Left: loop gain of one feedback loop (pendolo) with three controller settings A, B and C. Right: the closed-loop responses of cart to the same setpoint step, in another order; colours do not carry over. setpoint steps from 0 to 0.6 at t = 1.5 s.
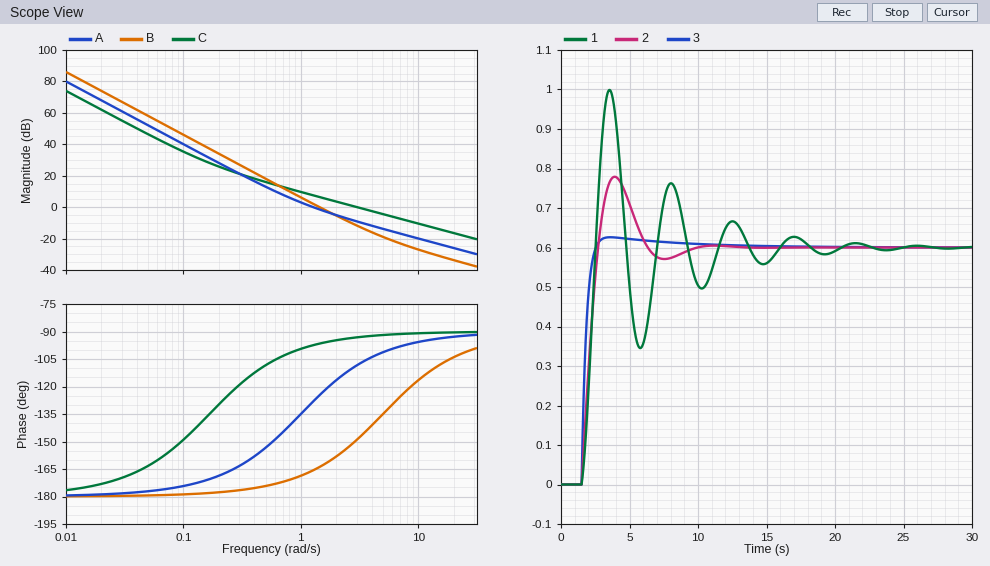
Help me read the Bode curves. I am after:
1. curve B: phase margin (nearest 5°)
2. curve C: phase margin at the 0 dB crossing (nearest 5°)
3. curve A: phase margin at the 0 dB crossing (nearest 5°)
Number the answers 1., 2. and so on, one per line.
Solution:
1. 15°
2. 85°
3. 50°
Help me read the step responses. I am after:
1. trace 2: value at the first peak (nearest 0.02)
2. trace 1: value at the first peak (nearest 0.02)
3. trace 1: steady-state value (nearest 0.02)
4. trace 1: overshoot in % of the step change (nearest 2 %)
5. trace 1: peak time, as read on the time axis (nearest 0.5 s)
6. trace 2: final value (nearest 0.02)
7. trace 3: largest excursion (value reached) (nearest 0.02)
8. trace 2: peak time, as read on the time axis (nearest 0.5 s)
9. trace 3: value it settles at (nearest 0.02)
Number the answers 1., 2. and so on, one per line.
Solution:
1. 0.78
2. 1.00
3. 0.60
4. 66 %
5. 3.5 s
6. 0.60
7. 0.62
8. 4.0 s
9. 0.60
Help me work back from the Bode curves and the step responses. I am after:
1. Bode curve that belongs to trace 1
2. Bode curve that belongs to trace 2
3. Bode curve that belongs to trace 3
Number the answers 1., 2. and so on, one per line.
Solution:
1. B
2. A
3. C
